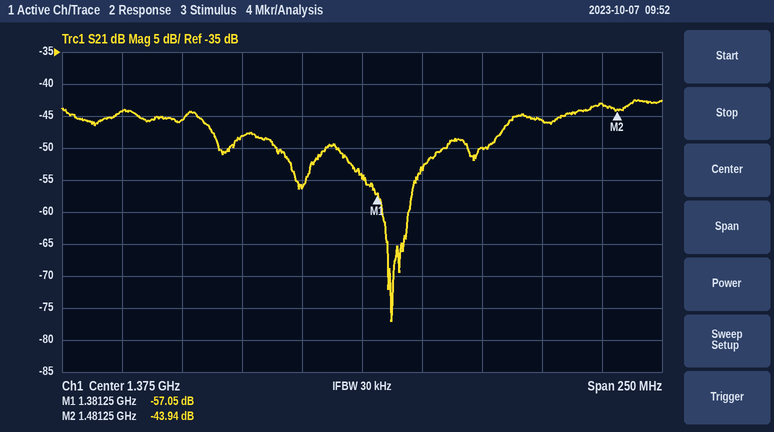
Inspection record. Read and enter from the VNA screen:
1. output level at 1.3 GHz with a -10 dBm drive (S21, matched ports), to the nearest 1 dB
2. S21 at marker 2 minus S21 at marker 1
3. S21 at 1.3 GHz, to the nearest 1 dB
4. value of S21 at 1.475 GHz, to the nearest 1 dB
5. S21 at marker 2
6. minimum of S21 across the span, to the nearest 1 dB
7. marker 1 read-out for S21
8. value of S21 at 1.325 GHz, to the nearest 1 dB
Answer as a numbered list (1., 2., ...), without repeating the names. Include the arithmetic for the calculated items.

1. -10 dBm + (-46 dB) = -56 dBm
2. -43.94 − (-57.05) = 13.11 dB
3. -46 dB
4. -43 dB
5. -43.94 dB
6. -77 dB
7. -57.05 dB
8. -48 dB
